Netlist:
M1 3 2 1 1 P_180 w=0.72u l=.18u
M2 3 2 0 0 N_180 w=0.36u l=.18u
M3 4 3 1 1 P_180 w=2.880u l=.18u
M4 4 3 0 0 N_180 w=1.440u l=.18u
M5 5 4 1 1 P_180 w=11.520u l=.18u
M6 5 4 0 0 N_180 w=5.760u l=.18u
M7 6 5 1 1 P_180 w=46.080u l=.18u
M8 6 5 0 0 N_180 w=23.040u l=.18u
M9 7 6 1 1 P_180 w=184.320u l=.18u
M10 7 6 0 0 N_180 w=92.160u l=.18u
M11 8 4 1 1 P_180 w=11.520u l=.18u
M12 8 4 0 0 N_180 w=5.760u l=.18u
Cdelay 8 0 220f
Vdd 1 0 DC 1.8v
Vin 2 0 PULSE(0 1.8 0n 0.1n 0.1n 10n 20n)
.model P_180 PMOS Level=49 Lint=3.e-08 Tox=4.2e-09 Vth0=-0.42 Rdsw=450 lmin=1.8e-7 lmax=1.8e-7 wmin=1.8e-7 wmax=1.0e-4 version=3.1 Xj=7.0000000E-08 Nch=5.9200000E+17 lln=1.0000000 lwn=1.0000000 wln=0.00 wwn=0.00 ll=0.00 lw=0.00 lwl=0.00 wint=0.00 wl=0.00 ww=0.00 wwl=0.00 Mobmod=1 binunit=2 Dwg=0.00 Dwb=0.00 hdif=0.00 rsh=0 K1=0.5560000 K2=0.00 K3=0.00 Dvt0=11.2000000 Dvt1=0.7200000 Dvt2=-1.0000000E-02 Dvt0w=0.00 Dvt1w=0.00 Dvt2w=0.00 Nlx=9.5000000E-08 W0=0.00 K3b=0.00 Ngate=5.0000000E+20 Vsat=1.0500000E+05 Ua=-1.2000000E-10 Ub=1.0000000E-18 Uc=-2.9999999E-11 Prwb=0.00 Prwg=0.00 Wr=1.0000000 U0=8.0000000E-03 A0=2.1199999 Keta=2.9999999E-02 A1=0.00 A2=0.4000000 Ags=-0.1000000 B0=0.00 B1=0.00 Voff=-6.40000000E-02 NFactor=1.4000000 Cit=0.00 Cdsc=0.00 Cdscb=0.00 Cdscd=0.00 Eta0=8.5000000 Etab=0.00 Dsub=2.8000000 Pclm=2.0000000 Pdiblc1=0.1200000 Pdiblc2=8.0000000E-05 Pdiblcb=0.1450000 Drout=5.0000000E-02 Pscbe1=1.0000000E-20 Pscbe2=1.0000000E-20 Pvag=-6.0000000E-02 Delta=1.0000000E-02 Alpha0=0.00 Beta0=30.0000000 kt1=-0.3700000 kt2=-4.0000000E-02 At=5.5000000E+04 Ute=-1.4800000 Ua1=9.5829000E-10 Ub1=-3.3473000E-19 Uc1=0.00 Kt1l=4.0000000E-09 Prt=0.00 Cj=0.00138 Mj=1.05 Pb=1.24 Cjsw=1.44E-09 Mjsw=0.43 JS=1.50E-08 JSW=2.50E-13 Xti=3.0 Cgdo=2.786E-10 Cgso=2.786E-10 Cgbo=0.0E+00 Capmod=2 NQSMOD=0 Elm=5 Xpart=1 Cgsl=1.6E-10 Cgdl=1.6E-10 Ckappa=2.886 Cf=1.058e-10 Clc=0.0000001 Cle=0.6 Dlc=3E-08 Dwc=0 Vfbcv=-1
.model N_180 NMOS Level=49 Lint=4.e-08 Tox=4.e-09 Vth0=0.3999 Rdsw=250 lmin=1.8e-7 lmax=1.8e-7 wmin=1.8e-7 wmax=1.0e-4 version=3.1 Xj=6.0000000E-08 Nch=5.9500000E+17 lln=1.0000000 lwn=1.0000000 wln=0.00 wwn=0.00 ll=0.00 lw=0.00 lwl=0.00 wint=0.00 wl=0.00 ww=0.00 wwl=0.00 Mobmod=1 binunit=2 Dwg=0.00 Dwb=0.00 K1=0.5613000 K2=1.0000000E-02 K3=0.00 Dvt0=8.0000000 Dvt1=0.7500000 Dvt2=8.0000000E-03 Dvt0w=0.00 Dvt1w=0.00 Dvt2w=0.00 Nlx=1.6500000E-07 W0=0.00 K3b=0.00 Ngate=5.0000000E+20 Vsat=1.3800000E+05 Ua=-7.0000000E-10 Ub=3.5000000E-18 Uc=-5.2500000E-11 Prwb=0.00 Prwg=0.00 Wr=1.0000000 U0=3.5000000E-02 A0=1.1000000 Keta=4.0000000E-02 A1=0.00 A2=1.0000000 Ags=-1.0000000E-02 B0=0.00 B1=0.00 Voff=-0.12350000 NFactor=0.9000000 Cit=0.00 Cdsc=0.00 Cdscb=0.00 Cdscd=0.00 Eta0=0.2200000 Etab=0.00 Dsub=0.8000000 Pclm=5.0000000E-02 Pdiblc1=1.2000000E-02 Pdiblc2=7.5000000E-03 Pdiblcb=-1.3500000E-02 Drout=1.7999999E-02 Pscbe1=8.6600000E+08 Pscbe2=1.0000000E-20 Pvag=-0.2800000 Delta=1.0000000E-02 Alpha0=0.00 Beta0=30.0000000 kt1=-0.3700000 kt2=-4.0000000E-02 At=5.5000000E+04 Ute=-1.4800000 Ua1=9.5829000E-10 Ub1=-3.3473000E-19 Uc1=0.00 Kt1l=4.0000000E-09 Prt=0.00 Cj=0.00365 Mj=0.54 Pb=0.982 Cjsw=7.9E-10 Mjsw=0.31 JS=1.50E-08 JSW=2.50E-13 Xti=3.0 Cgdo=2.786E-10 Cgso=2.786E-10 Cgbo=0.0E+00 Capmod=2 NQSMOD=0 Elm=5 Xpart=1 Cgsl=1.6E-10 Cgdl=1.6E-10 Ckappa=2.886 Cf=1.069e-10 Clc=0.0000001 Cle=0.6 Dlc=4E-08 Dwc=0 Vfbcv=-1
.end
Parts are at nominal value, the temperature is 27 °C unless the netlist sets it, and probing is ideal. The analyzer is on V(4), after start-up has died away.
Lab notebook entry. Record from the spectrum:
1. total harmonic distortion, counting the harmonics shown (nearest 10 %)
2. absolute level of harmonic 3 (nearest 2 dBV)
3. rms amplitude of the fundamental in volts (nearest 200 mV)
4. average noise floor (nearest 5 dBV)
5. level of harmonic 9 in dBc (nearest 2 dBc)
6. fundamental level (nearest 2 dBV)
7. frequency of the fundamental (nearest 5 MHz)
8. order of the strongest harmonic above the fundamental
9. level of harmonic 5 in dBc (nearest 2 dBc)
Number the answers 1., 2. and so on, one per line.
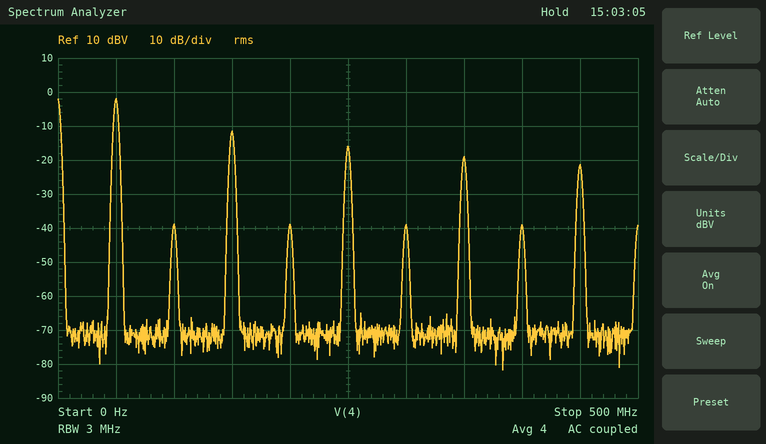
1. 40 %
2. -12 dBV
3. 800 mV
4. -70 dBV
5. -20 dBc
6. -2 dBV
7. 50 MHz
8. 3
9. -14 dBc
